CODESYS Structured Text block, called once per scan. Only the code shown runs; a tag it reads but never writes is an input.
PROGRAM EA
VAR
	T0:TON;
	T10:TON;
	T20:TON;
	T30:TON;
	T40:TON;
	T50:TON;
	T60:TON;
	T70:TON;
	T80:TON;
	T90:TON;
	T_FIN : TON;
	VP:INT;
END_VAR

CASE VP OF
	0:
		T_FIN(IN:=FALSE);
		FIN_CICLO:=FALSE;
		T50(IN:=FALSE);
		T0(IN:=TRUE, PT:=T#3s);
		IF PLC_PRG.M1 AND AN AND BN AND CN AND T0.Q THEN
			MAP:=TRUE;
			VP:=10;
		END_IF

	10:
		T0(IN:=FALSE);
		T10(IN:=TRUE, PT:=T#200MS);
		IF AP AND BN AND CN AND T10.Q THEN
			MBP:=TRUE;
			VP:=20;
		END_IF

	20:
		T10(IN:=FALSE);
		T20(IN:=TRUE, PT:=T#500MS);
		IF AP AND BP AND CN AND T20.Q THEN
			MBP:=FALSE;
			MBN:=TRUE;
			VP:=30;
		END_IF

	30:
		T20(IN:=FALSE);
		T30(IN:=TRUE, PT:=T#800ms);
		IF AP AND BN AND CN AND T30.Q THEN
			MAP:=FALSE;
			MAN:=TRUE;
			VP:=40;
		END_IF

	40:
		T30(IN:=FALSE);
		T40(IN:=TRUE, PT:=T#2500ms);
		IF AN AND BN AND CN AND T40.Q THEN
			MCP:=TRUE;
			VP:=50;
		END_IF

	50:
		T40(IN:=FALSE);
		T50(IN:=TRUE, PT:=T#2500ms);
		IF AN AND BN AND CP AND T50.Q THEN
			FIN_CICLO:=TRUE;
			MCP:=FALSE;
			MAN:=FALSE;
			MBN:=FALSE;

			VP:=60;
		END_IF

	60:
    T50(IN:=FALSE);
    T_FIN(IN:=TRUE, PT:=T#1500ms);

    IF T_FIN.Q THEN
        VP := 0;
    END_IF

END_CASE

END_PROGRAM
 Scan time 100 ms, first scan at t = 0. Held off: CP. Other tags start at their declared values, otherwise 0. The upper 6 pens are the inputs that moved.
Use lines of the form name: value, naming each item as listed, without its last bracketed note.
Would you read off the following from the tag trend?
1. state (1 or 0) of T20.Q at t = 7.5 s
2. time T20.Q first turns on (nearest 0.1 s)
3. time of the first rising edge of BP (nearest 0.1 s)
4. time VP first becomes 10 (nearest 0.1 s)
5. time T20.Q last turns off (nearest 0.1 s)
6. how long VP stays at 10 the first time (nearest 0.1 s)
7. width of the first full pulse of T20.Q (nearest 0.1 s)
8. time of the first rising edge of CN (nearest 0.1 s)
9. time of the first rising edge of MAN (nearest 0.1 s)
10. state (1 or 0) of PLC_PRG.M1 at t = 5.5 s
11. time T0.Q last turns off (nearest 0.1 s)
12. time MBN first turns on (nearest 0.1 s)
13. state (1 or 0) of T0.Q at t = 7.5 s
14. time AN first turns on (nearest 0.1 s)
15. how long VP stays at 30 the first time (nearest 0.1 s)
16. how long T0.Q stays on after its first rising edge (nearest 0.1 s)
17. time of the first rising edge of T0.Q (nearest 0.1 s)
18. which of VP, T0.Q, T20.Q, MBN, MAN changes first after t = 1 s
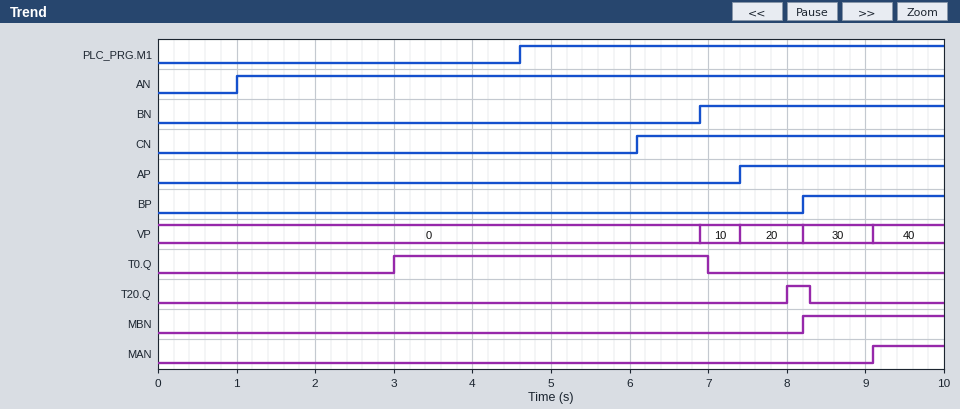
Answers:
state (1 or 0) of T20.Q at t = 7.5 s: 0
time T20.Q first turns on: 8.0 s
time of the first rising edge of BP: 8.2 s
time VP first becomes 10: 6.9 s
time T20.Q last turns off: 8.3 s
how long VP stays at 10 the first time: 0.5 s
width of the first full pulse of T20.Q: 0.3 s
time of the first rising edge of CN: 6.1 s
time of the first rising edge of MAN: 9.1 s
state (1 or 0) of PLC_PRG.M1 at t = 5.5 s: 1
time T0.Q last turns off: 7.0 s
time MBN first turns on: 8.2 s
state (1 or 0) of T0.Q at t = 7.5 s: 0
time AN first turns on: 1.0 s
how long VP stays at 30 the first time: 0.9 s
how long T0.Q stays on after its first rising edge: 4.0 s
time of the first rising edge of T0.Q: 3.0 s
which of VP, T0.Q, T20.Q, MBN, MAN changes first after t = 1 s: T0.Q
